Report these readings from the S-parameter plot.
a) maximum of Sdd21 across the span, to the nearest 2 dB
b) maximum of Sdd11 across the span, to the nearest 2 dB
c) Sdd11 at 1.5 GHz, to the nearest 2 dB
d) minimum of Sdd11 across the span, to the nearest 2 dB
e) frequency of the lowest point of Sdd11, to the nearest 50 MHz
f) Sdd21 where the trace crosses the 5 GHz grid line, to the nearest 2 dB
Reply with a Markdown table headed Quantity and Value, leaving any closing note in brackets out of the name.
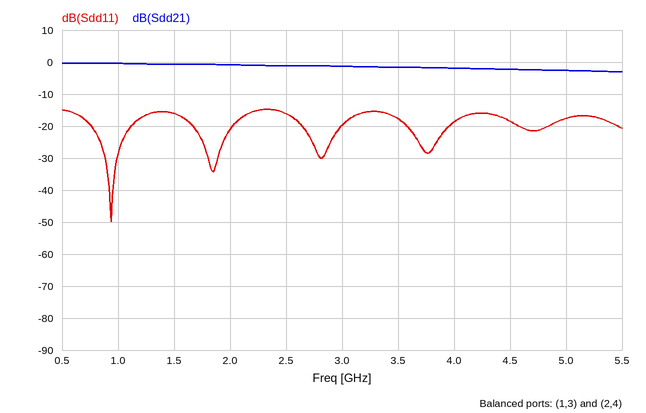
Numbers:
| Quantity | Value |
|---|---|
| maximum of Sdd21 across the span, to the nearest 2 dB | 0 dB |
| maximum of Sdd11 across the span, to the nearest 2 dB | -14 dB |
| Sdd11 at 1.5 GHz, to the nearest 2 dB | -16 dB |
| minimum of Sdd11 across the span, to the nearest 2 dB | -50 dB |
| frequency of the lowest point of Sdd11, to the nearest 50 MHz | 950 MHz |
| Sdd21 where the trace crosses the 5 GHz grid line, to the nearest 2 dB | -2 dB |
